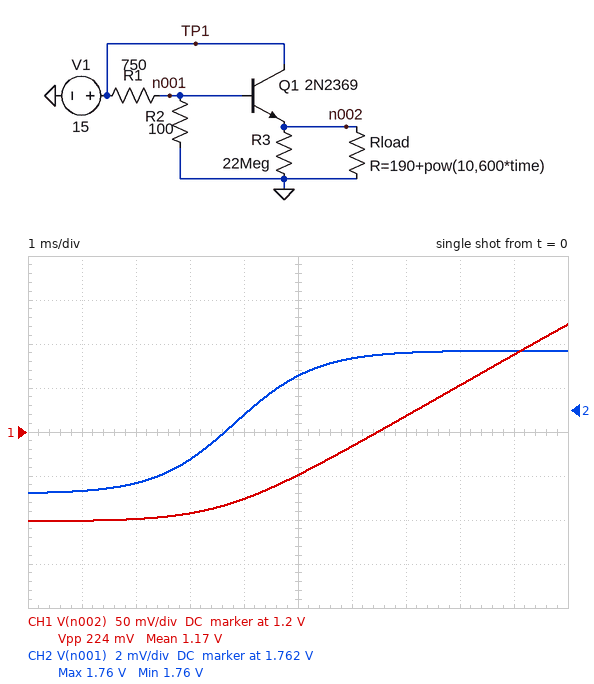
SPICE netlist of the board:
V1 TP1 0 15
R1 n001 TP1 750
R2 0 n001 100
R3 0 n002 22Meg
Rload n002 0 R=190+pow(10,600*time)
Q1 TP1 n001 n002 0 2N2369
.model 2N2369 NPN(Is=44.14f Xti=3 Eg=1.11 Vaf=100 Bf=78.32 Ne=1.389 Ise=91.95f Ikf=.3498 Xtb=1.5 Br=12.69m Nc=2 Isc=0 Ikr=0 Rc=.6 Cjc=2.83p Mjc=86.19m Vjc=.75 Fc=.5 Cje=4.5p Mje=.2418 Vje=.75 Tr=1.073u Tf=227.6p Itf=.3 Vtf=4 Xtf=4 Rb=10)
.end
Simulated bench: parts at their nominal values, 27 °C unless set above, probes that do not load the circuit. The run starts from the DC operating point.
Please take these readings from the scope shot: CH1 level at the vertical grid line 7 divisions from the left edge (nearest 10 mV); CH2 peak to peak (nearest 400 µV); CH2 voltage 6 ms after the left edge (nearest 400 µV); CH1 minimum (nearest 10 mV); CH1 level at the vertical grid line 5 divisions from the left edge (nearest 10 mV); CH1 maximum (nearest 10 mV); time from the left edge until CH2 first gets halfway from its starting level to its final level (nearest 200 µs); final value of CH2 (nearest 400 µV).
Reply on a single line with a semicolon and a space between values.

1.22 V; 6.4 mV; 1.7644 V; 1.10 V; 1.15 V; 1.32 V; 3.8 ms; 1.7648 V
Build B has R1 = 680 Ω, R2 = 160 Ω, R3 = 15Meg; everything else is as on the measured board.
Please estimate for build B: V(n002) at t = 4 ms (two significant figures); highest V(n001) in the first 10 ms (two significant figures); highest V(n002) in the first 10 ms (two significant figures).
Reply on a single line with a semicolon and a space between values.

2.2 V; 2.9 V; 2.4 V
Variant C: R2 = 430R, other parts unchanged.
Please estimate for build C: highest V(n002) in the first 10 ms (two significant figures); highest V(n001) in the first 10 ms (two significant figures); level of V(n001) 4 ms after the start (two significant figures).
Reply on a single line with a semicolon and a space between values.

5.0 V; 5.5 V; 5.4 V
